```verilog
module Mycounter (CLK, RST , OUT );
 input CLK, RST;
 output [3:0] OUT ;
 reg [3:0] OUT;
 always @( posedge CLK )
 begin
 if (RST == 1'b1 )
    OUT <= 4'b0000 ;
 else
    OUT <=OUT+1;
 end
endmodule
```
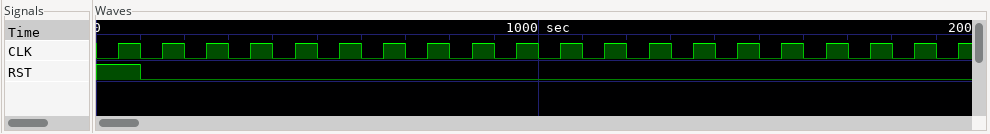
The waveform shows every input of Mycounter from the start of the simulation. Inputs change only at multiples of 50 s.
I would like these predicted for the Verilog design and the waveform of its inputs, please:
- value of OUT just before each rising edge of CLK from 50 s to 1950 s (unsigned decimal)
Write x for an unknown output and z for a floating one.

x, 0, 1, 2, 3, 4, 5, 6, 7, 8, 9, 10, 11, 12, 13, 14, 15, 0, 1, 2
